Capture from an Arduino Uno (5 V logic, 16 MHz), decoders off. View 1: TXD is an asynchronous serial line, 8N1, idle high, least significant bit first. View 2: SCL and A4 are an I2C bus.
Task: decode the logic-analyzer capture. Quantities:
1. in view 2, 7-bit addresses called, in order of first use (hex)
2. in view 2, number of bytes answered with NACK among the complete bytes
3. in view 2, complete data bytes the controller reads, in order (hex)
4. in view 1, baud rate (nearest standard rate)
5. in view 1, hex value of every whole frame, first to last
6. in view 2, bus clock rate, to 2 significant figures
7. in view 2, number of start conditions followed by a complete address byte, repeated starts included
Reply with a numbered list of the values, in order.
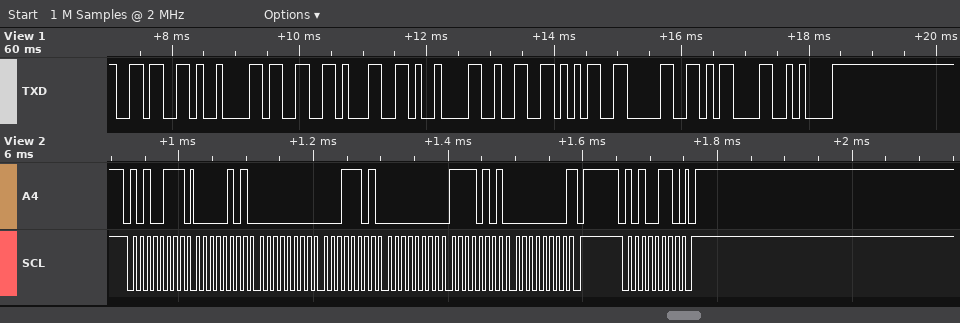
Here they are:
1. 0x53
2. 1
3. 05 00 1D 00 F5 00
4. 9600 baud
5. 36 09 33 31 09 32 35 30 0D 0A
6. 100 kHz
7. 2
